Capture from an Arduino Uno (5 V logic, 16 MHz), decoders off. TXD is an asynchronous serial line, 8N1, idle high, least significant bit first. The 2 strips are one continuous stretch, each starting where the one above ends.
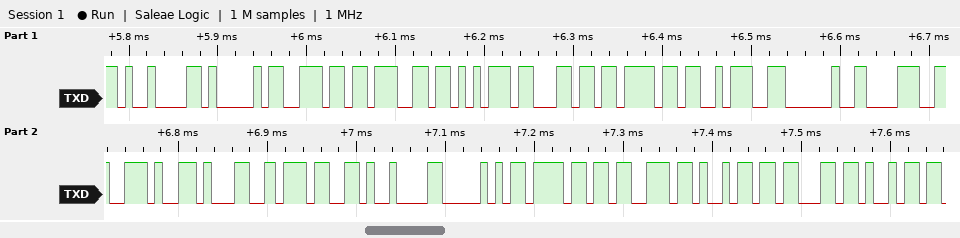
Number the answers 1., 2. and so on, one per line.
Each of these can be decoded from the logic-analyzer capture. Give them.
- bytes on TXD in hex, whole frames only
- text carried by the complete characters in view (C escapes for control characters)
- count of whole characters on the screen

1. 09 41 6E 67 75 6C 6F 3A 20 38 2E 31 37 09 50 6F 73 69 63 69
2. "\tAngulo: 8.17\tPosici"
3. 20
